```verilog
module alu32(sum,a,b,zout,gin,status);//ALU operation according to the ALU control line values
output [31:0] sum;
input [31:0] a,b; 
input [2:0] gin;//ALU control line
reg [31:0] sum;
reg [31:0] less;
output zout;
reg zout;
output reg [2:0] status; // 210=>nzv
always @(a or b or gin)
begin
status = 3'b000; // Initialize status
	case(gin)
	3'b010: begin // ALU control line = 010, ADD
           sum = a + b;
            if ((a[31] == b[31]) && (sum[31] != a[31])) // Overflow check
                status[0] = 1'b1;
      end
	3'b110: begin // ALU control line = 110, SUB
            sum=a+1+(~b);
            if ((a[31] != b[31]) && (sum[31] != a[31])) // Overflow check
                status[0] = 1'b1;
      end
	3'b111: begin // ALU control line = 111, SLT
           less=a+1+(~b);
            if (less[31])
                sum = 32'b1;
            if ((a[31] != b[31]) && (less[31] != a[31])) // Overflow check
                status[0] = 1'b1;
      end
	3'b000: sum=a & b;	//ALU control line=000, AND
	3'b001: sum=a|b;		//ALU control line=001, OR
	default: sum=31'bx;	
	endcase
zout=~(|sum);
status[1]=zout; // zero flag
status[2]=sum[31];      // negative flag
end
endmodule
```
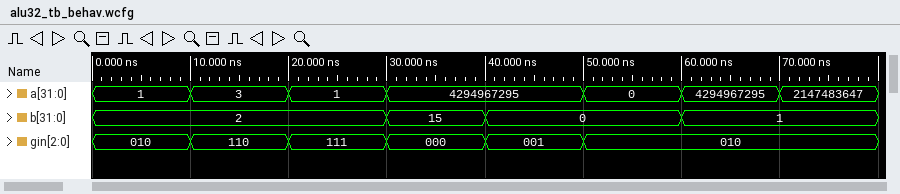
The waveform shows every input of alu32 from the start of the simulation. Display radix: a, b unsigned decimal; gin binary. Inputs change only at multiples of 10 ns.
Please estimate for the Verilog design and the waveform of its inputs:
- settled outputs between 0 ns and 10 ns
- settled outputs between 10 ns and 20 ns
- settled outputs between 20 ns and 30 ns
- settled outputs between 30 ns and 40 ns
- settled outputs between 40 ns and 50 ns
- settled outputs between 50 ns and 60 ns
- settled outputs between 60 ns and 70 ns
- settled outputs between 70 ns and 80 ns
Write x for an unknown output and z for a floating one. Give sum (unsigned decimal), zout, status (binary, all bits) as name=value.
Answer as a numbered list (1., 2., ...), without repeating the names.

1. sum=3, zout=0, status=000
2. sum=1, zout=0, status=000
3. sum=1, zout=0, status=000
4. sum=15, zout=0, status=000
5. sum=4294967295, zout=0, status=100
6. sum=0, zout=1, status=010
7. sum=0, zout=1, status=010
8. sum=2147483648, zout=0, status=101
